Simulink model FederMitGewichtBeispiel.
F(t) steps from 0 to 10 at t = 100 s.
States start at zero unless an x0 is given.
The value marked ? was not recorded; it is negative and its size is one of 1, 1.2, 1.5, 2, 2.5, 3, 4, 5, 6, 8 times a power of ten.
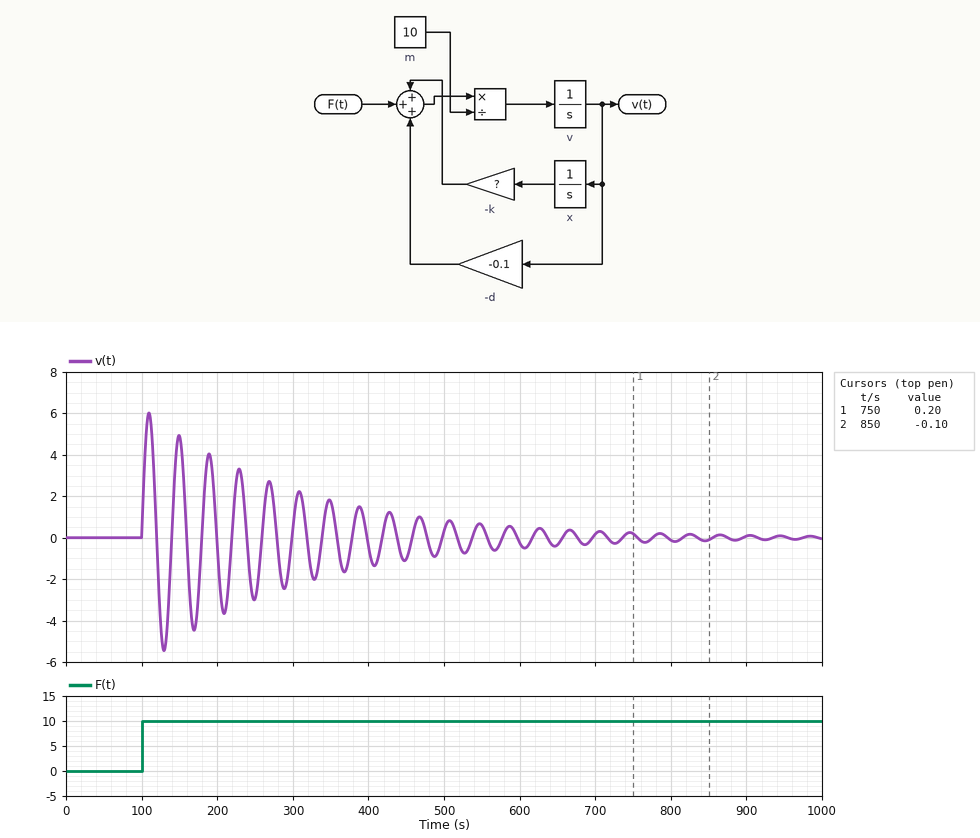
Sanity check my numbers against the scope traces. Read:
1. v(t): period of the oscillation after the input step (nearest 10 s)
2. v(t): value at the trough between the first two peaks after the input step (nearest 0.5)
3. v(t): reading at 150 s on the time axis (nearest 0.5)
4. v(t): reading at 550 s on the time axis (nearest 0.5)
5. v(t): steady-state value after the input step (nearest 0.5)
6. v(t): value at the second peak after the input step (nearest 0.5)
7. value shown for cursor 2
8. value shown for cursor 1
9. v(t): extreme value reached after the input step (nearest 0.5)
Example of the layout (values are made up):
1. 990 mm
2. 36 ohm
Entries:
1. 40 s
2. -5.5
3. 5.0
4. 0.5
5. 0.0
6. 5.0
7. -0.10
8. 0.20
9. 6.0
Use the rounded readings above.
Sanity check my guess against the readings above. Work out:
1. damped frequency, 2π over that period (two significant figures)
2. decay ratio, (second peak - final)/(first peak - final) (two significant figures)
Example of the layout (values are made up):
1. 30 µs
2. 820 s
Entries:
1. 0.16 rad/s
2. 0.83
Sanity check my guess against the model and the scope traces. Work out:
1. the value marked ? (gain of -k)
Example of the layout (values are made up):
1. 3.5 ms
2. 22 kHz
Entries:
1. -0.25
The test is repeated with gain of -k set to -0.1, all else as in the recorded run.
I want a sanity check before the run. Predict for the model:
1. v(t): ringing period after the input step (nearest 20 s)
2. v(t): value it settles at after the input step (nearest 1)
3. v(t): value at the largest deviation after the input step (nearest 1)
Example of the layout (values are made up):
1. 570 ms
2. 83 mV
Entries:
1. 60 s
2. 0
3. 9
